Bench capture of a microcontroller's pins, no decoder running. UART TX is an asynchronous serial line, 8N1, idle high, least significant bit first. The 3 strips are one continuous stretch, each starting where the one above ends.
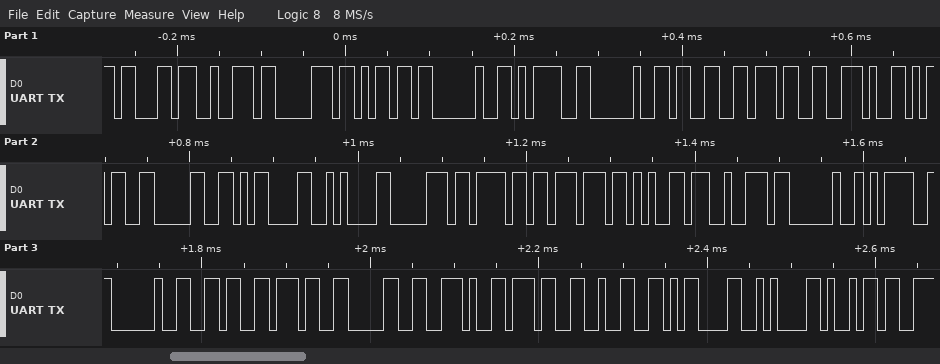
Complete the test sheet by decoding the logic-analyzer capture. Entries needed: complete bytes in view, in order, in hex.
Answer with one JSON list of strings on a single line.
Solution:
["63 72 70 6D 20 3D 20 33 37 2E 35 30 0D 0A 70 6F 77 65 72 20 3D 20 36 37 30 2E 37 32 0D 0A 69"]
